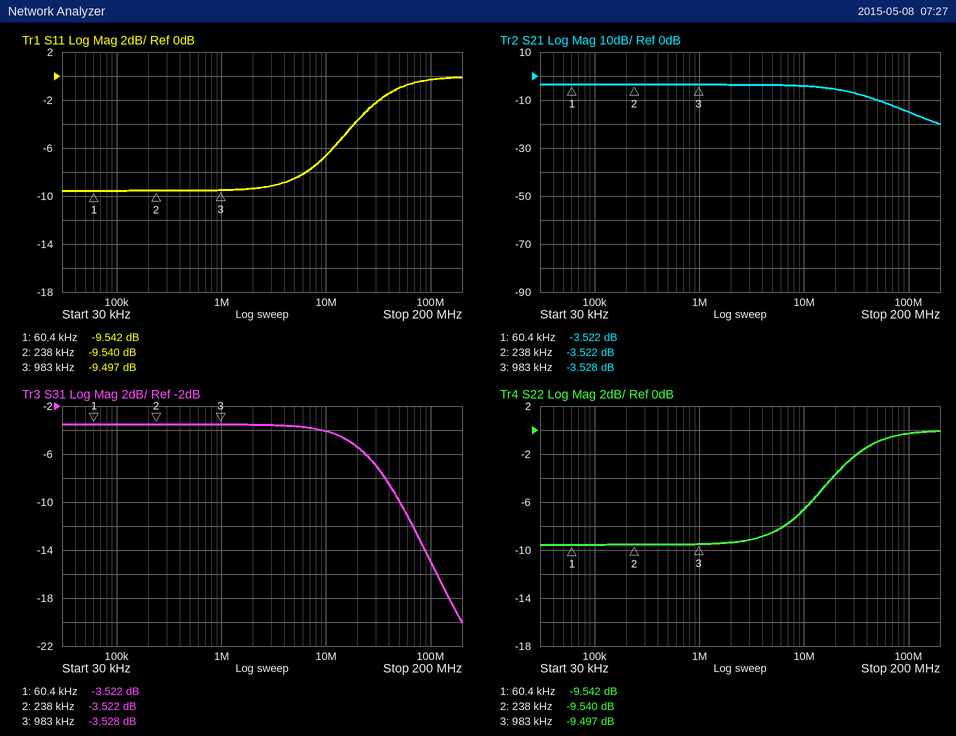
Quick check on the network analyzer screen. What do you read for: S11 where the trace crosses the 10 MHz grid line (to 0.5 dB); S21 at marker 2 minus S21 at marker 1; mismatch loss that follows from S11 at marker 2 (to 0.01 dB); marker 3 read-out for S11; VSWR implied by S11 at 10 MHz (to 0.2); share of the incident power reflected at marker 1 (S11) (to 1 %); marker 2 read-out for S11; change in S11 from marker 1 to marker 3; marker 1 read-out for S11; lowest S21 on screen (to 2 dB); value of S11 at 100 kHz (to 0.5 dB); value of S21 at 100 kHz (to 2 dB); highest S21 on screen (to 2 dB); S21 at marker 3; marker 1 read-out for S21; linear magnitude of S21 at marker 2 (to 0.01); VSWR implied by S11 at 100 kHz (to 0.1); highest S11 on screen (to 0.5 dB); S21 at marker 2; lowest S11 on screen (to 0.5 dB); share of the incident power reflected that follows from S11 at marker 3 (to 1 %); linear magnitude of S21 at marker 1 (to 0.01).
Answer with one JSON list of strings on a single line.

["-6.5 dB", "0.000 dB", "0.51 dB", "-9.497 dB", "2.8", "11 %", "-9.540 dB", "0.045 dB", "-9.542 dB", "-20 dB", "-9.5 dB", "-4 dB", "-4 dB", "-3.528 dB", "-3.522 dB", "0.67", "2.0", "0.0 dB", "-3.522 dB", "-9.5 dB", "11 %", "0.67"]
